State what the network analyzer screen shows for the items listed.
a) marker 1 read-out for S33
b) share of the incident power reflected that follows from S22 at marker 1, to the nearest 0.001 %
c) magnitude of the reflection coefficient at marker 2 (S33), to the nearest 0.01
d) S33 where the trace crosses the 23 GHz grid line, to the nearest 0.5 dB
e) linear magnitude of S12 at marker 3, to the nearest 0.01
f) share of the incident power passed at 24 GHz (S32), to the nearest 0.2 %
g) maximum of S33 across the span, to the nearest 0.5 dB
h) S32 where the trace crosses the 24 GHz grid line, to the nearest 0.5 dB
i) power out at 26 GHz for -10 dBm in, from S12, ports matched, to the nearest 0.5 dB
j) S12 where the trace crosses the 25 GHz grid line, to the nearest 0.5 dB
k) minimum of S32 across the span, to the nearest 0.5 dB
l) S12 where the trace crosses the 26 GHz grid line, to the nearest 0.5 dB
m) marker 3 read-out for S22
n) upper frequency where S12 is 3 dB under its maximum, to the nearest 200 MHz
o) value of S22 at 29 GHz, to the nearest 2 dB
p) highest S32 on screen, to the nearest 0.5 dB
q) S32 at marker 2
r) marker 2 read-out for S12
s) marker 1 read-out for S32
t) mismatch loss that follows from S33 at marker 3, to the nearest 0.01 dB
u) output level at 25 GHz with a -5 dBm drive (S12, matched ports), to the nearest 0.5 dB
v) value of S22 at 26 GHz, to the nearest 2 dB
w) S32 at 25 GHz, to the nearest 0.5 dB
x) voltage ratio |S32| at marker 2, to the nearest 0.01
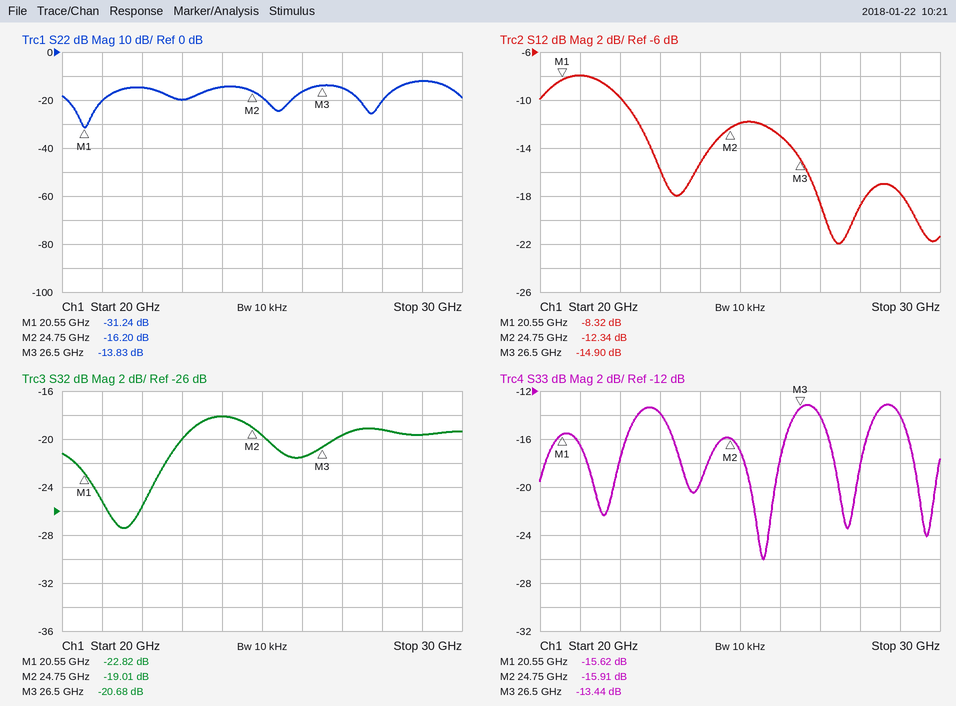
-15.62 dB
0.075 %
0.16
-14.0 dB
0.18
1.6 %
-13.0 dB
-18.0 dB
-23.0 dBm
-12.0 dB
-27.5 dB
-13.0 dB
-13.83 dB
22.2 GHz
-12 dB
-18.0 dB
-19.01 dB
-12.34 dB
-22.82 dB
0.20 dB
-17.0 dBm
-16 dB
-19.5 dB
0.11
